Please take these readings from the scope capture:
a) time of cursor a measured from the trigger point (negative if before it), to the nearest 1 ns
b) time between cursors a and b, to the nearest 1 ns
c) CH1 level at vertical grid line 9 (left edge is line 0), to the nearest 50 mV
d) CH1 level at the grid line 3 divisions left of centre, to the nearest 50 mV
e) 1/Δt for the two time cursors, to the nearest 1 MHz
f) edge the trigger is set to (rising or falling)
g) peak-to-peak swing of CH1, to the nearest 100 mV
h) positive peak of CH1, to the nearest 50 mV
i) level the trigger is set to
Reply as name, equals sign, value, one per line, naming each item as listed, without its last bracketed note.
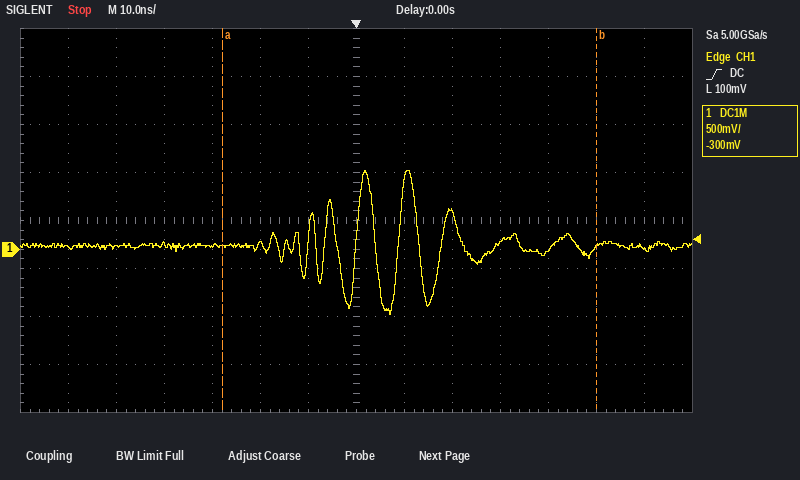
time of cursor a measured from the trigger point (negative if before it), to the nearest 1 ns = -28 ns
time between cursors a and b, to the nearest 1 ns = 78 ns
CH1 level at vertical grid line 9 (left edge is line 0), to the nearest 50 mV = 400 mV
CH1 level at the grid line 3 divisions left of centre, to the nearest 50 mV = 50 mV
1/Δt for the two time cursors, to the nearest 1 MHz = 13 MHz
edge the trigger is set to = rising
peak-to-peak swing of CH1, to the nearest 100 mV = 1.50 V
positive peak of CH1, to the nearest 50 mV = 800 mV
level the trigger is set to = 100 mV
